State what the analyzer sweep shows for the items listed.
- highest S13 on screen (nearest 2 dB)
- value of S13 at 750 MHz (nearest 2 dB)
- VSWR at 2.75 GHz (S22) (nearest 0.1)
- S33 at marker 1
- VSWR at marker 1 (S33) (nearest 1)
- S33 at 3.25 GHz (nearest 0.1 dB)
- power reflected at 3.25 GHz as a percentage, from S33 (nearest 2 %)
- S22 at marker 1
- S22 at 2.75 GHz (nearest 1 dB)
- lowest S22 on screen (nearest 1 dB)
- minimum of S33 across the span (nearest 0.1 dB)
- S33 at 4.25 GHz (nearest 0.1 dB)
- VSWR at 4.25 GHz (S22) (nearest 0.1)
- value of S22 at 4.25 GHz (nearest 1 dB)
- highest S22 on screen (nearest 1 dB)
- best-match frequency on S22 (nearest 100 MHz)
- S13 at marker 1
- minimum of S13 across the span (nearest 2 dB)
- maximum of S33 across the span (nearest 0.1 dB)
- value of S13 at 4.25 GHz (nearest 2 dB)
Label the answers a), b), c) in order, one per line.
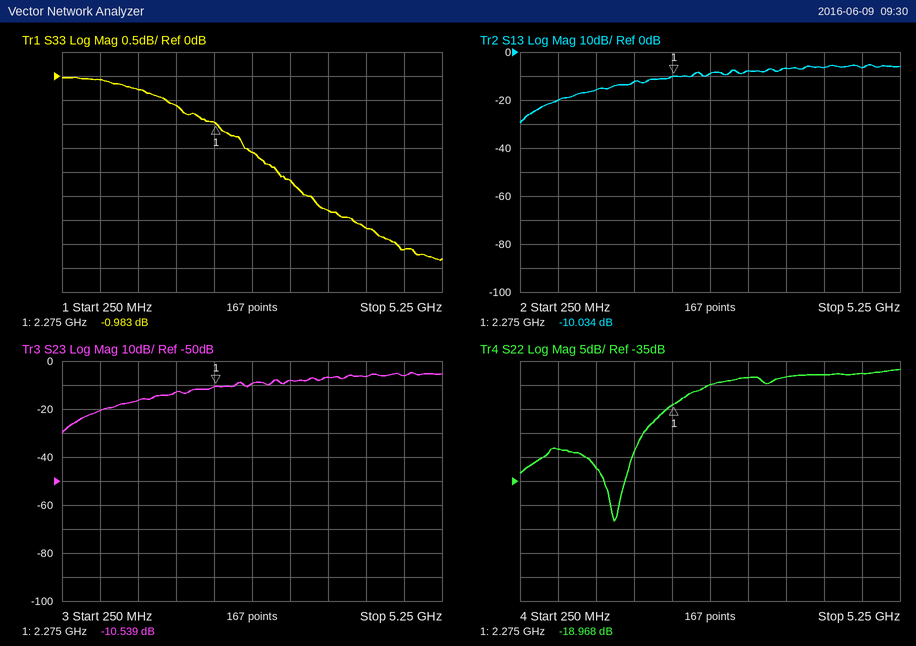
a) -6 dB
b) -20 dB
c) 1.4
d) -0.983 dB
e) 18
f) -2.2 dB
g) 60 %
h) -18.968 dB
i) -15 dB
j) -43 dB
k) -3.8 dB
l) -3.2 dB
m) 1.6
n) -13 dB
o) -12 dB
p) 1.5 GHz
q) -10.034 dB
r) -30 dB
s) 0.0 dB
t) -6 dB
